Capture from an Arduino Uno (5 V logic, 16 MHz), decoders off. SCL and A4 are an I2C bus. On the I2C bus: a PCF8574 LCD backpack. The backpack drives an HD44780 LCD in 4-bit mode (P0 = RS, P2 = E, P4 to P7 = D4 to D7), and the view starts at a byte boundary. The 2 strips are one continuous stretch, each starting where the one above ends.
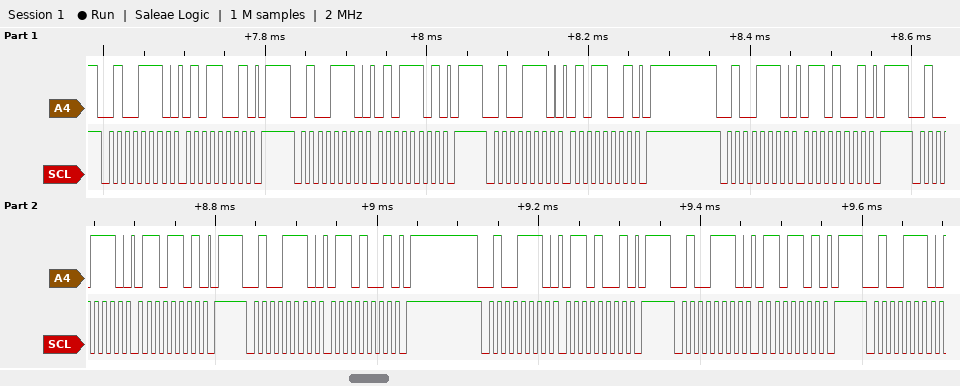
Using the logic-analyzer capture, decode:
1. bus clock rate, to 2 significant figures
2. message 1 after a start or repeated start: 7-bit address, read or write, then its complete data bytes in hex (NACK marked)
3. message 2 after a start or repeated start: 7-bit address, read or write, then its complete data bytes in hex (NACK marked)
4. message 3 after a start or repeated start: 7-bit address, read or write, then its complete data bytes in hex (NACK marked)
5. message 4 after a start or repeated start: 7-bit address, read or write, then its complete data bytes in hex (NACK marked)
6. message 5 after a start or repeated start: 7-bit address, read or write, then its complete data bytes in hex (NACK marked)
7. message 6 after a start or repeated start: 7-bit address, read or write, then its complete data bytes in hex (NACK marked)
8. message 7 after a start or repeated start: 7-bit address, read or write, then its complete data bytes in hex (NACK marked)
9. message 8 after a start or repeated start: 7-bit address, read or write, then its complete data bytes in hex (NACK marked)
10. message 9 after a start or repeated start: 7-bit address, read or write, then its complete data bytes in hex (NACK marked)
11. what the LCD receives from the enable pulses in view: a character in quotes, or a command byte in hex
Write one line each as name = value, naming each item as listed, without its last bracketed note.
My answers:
bus clock rate, to 2 significant figures = 100 kHz
message 1 after a start or repeated start: 7-bit address, read or write, then its complete data bytes in hex = 0x27 write: 59
message 2 after a start or repeated start: 7-bit address, read or write, then its complete data bytes in hex = 0x27 write: 5D
message 3 after a start or repeated start: 7-bit address, read or write, then its complete data bytes in hex = 0x27 write: 59
message 4 after a start or repeated start: 7-bit address, read or write, then its complete data bytes in hex = 0x27 write: 69
message 5 after a start or repeated start: 7-bit address, read or write, then its complete data bytes in hex = 0x27 write: 6D
message 6 after a start or repeated start: 7-bit address, read or write, then its complete data bytes in hex = 0x27 write: 69
message 7 after a start or repeated start: 7-bit address, read or write, then its complete data bytes in hex = 0x27 write: 69
message 8 after a start or repeated start: 7-bit address, read or write, then its complete data bytes in hex = 0x27 write: 6D
message 9 after a start or repeated start: 7-bit address, read or write, then its complete data bytes in hex = 0x27 write
what the LCD receives from the enable pulses in view: a character in quotes, or a command byte in hex = 'V'
